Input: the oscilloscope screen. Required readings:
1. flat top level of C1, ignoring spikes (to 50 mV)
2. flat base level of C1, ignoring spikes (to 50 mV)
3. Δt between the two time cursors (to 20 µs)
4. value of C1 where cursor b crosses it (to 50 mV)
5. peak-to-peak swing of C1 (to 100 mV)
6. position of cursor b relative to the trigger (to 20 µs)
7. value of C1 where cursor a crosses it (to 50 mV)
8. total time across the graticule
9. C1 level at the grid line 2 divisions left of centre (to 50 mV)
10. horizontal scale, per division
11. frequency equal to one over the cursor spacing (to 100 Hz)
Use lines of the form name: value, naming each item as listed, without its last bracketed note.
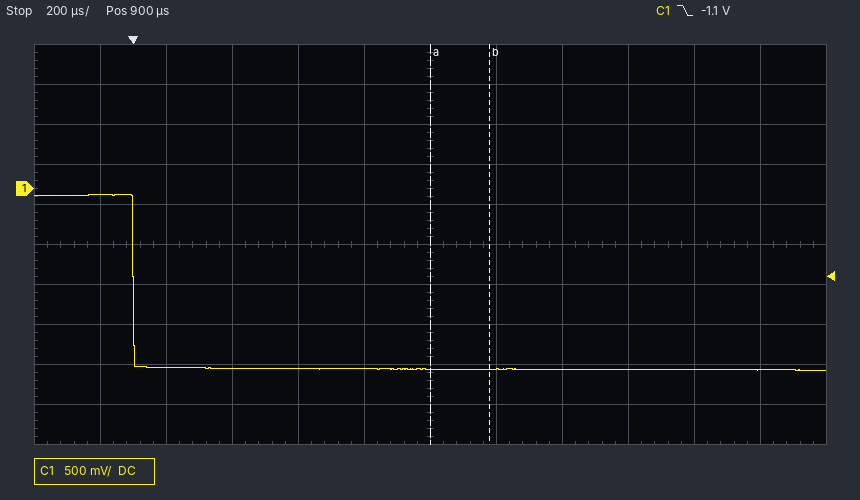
flat top level of C1, ignoring spikes: -100 mV
flat base level of C1, ignoring spikes: -2.25 V
Δt between the two time cursors: 180 µs
value of C1 where cursor b crosses it: -2.25 V
peak-to-peak swing of C1: 2.20 V
position of cursor b relative to the trigger: +1.08 ms
value of C1 where cursor a crosses it: -2.25 V
total time across the graticule: 2.4 ms
C1 level at the grid line 2 divisions left of centre: -2.25 V
horizontal scale, per division: 200 µs
frequency equal to one over the cursor spacing: 5.6 kHz
